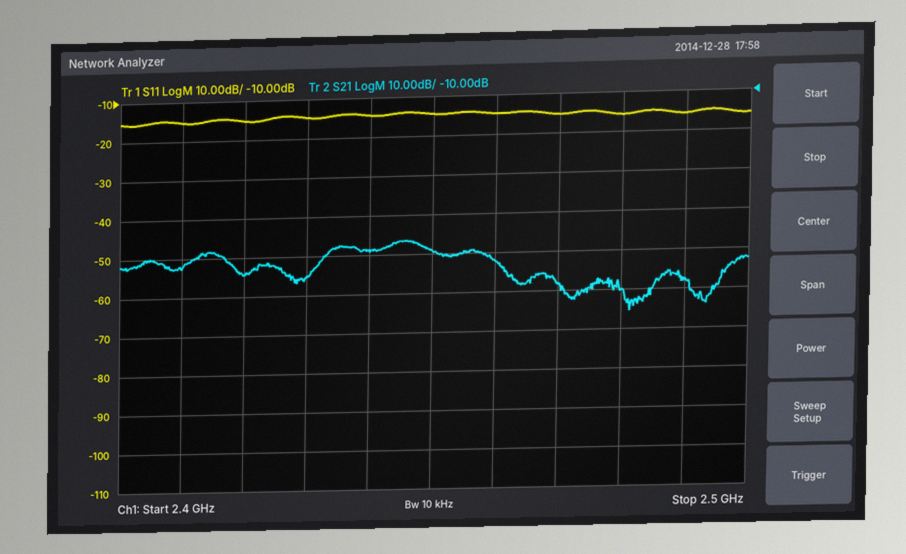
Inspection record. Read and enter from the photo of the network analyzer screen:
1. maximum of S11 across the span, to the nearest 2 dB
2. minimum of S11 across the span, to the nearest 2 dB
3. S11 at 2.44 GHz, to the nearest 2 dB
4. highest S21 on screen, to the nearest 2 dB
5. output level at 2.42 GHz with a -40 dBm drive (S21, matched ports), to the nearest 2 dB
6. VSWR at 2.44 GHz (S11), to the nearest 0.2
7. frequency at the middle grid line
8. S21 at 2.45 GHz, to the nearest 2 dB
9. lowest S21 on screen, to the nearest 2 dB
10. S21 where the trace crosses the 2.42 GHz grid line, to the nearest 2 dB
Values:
-14 dB
-16 dB
-14 dB
-46 dB
-94 dBm
1.4
2.45 GHz
-50 dB
-66 dB
-54 dB
